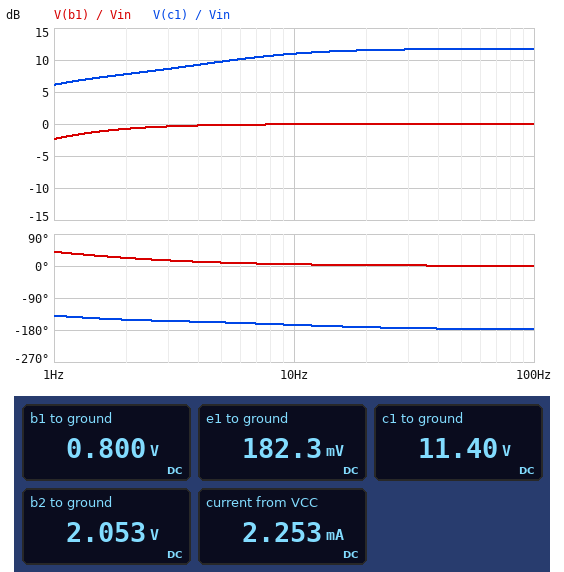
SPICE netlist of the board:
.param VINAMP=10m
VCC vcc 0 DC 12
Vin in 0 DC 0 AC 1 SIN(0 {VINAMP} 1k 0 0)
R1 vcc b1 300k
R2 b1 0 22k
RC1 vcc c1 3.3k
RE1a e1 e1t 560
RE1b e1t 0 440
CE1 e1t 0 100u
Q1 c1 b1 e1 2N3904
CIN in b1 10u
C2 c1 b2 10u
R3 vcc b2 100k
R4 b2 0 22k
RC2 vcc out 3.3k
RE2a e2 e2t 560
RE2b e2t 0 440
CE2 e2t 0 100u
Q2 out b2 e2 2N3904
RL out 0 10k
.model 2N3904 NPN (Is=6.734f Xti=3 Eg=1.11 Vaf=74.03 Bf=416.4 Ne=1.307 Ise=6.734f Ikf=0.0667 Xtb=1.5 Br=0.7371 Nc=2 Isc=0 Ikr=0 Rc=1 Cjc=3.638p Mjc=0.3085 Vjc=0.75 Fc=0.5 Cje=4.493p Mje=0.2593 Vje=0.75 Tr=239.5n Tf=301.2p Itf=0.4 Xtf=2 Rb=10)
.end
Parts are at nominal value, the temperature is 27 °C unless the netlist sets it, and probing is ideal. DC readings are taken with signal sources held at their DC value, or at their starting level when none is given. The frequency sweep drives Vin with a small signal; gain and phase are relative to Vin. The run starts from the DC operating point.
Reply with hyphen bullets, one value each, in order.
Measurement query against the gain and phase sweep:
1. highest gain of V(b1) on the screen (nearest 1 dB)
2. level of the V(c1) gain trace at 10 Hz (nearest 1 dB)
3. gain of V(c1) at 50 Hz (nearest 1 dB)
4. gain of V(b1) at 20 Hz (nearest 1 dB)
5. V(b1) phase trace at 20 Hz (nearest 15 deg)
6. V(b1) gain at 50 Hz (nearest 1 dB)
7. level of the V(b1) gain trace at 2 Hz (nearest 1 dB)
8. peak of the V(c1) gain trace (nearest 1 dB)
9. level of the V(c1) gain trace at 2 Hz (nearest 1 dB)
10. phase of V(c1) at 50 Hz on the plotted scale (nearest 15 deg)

- 0 dB
- 11 dB
- 12 dB
- 0 dB
- 0 deg
- 0 dB
- -1 dB
- 12 dB
- 8 dB
- -180 deg
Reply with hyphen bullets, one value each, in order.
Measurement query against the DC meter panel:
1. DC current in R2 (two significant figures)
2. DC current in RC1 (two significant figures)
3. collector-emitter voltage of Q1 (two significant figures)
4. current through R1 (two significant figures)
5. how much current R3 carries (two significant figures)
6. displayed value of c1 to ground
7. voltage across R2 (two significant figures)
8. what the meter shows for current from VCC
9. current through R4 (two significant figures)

- 36 µA
- 180 µA
- 11 V
- 37 µA
- 99 µA
- 11.40 V
- 800 mV
- 2.253 mA
- 93 µA
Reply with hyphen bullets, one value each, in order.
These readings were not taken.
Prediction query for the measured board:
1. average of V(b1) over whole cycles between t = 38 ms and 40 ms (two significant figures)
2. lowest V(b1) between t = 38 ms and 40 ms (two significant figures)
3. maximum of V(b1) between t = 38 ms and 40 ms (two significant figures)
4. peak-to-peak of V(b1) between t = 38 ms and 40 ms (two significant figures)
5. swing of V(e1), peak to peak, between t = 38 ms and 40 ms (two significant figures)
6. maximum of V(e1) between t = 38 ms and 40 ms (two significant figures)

- 800 mV
- 790 mV
- 810 mV
- 20 mV
- 16 mV
- 190 mV
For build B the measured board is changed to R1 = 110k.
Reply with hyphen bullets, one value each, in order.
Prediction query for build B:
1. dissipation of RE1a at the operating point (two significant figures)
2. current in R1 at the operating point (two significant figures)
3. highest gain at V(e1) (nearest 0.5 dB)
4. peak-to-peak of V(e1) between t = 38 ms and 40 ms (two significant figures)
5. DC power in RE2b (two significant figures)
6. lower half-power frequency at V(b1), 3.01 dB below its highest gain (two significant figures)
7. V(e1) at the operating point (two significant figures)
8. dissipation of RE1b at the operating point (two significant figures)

- 850 µW
- 92 µA
- -0.5 dB
- 19 mV
- 840 µW
- 940 mHz
- 1.2 V
- 670 µW
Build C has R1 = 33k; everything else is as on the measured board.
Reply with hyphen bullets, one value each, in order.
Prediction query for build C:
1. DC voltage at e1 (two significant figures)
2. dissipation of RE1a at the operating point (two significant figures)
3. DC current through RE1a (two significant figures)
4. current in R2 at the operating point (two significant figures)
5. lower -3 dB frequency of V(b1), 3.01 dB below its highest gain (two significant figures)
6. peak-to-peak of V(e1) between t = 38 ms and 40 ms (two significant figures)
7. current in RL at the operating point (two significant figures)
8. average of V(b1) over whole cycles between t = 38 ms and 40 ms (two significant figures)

- 2.8 V
- 4.5 mW
- 2.8 mA
- 160 µA
- 32 Hz
- 19 mV
- 560 µA
- 3.5 V
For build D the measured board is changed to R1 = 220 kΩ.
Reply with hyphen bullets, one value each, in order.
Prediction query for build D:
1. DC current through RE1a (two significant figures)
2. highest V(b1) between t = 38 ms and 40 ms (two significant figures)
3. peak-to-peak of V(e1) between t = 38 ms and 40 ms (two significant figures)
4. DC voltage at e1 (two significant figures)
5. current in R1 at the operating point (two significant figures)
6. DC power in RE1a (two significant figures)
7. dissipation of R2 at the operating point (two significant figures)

- 410 µA
- 1.1 V
- 18 mV
- 410 mV
- 50 µA
- 95 µW
- 50 µW
